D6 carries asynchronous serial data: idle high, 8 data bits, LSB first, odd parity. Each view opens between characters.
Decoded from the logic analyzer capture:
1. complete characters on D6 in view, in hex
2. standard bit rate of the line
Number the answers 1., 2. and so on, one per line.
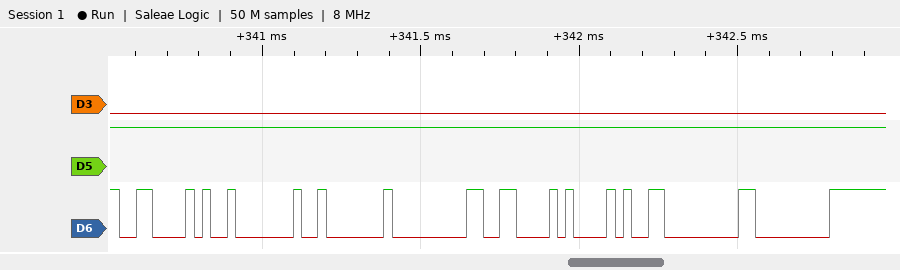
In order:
1. 86, 02, 02, 00, 86, 28, 00, 00
2. 38400 baud
